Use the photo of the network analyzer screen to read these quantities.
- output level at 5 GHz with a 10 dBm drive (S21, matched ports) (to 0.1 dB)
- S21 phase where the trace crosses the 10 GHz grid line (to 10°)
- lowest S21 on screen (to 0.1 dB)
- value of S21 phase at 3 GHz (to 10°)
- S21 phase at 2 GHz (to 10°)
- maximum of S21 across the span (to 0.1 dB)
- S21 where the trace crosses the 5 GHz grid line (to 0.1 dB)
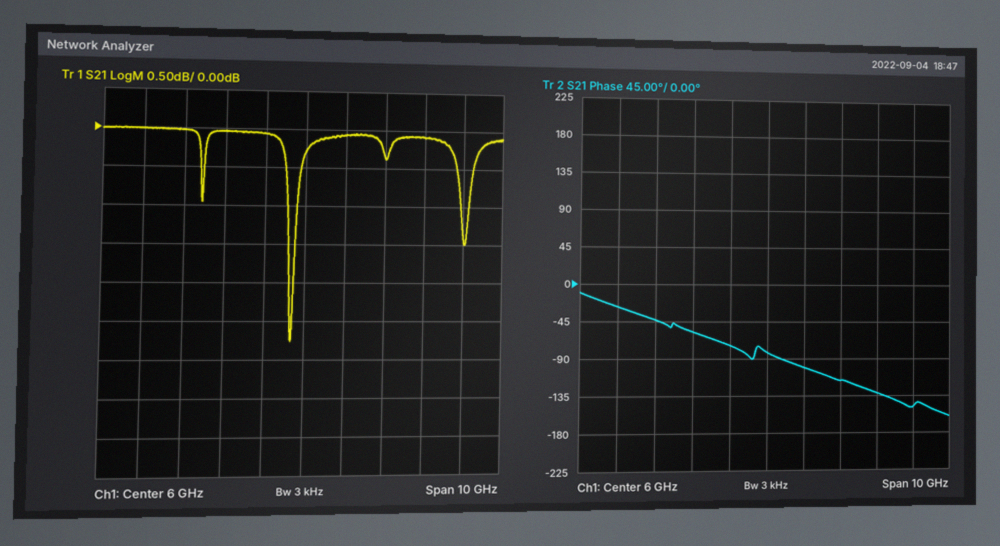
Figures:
9.9 dBm
-150°
-2.8 dB
-40°
-30°
0.0 dB
-0.1 dB
